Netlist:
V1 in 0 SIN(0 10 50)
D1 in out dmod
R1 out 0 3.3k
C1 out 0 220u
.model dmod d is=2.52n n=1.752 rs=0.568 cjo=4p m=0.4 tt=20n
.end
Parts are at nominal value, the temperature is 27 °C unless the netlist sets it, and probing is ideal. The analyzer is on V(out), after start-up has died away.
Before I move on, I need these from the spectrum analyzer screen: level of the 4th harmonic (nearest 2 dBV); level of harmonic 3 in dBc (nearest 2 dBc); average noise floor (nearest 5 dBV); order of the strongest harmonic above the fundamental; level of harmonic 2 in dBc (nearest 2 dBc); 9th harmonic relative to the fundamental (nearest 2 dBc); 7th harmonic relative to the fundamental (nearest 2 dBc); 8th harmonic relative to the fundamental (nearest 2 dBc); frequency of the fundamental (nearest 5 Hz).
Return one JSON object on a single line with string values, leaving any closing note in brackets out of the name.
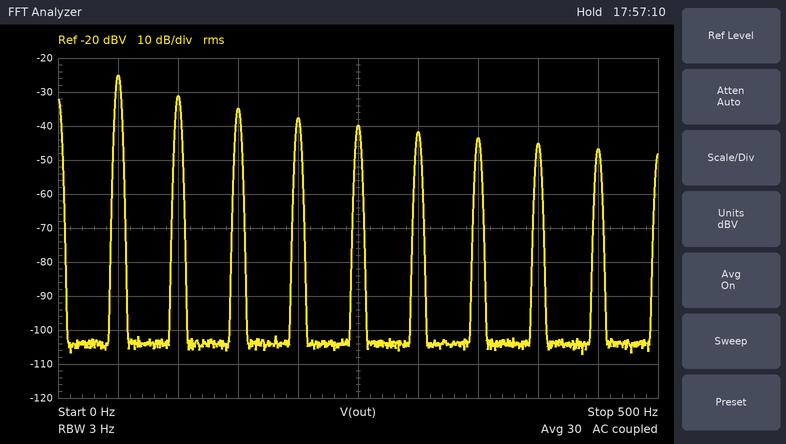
{"level of the 4th harmonic": "-38 dBV", "level of harmonic 3 in dBc": "-10 dBc", "average noise floor": "-105 dBV", "order of the strongest harmonic above the fundamental": "2", "level of harmonic 2 in dBc": "-6 dBc", "9th harmonic relative to the fundamental": "-22 dBc", "7th harmonic relative to the fundamental": "-18 dBc", "8th harmonic relative to the fundamental": "-20 dBc", "frequency of the fundamental": "50 Hz"}
